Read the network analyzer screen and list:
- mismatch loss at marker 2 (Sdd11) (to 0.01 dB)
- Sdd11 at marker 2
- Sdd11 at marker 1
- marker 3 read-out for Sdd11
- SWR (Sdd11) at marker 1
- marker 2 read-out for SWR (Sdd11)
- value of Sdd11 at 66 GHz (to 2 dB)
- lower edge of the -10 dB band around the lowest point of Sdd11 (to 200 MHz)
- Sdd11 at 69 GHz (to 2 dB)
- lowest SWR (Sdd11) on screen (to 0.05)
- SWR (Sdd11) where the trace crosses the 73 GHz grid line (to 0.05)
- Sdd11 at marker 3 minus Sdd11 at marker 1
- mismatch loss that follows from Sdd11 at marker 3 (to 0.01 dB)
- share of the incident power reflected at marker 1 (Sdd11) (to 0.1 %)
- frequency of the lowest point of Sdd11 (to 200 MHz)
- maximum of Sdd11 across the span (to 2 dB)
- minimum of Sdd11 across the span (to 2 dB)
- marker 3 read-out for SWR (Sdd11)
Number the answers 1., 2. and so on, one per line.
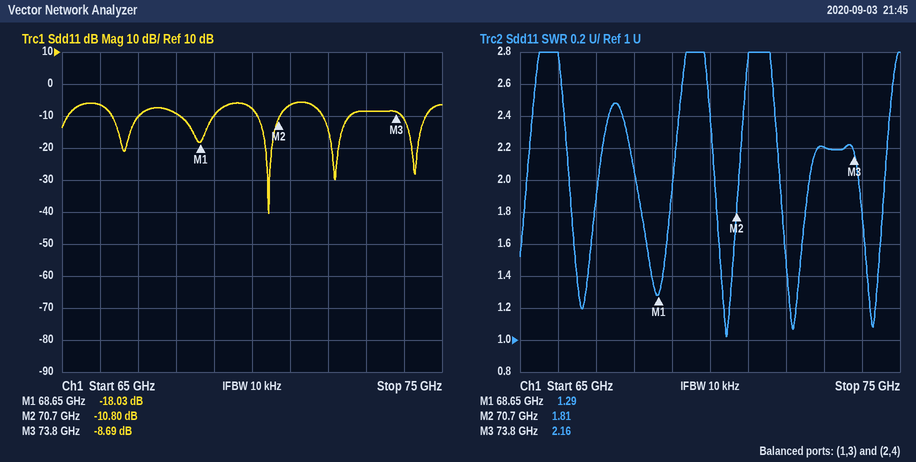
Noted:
1. 0.38 dB
2. -10.80 dB
3. -18.03 dB
4. -8.69 dB
5. 1.29
6. 1.81
7. -6 dB
8. 70.2 GHz
9. -10 dB
10. 1.00
11. 2.20
12. 9.34 dB
13. 0.63 dB
14. 1.6 %
15. 70.4 GHz
16. -6 dB
17. -40 dB
18. 2.16
